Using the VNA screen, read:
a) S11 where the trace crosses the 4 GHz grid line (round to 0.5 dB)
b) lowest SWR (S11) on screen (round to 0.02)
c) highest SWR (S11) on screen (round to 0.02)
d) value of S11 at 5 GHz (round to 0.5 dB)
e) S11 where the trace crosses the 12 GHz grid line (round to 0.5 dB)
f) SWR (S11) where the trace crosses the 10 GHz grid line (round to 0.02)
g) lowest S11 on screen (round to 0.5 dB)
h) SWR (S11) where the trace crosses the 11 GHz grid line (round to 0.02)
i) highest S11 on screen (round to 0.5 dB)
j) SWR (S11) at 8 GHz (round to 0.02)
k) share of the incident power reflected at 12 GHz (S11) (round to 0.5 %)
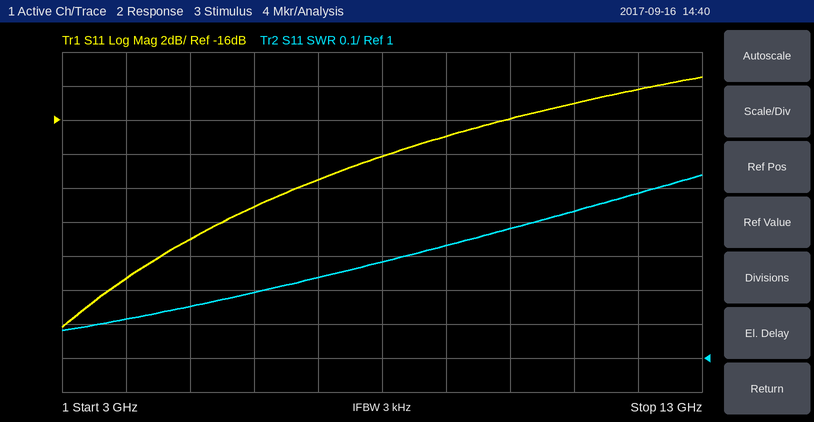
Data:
-25.5 dB
1.08
1.54
-23.0 dB
-14.0 dB
1.38
-28.0 dB
1.44
-13.5 dB
1.28
4.0 %
